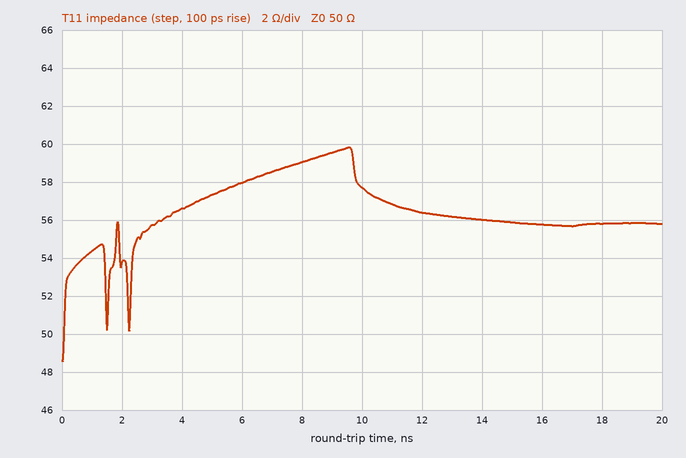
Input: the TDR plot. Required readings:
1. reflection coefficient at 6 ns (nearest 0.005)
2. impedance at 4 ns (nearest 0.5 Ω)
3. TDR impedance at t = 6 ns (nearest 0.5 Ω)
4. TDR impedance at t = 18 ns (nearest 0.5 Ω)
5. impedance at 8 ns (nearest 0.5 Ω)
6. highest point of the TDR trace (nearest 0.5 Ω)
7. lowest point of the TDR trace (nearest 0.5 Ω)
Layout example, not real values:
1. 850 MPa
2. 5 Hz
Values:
1. +0.075
2. 56.5 Ω
3. 58.0 Ω
4. 56.0 Ω
5. 59.0 Ω
6. 60.0 Ω
7. 48.5 Ω
